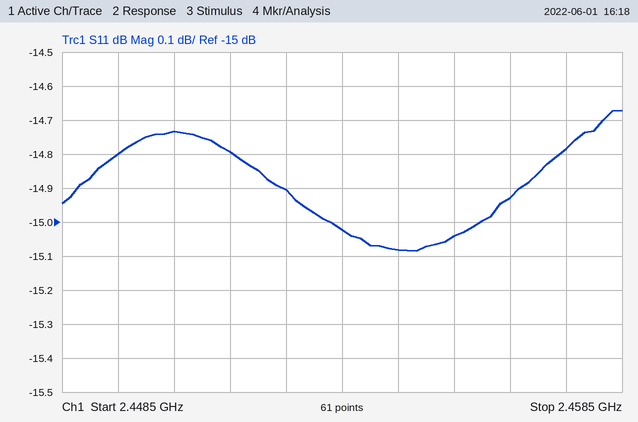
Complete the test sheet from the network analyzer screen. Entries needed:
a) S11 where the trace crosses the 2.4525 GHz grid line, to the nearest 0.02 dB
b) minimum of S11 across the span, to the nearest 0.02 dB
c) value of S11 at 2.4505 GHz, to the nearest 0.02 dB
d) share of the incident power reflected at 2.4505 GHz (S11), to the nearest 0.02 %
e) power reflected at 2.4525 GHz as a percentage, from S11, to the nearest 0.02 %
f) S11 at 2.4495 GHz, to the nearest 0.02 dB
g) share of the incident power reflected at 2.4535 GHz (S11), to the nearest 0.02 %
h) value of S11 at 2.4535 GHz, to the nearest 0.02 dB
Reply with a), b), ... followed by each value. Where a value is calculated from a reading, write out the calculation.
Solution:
a) -14.90 dB
b) -15.08 dB
c) -14.74 dB
d) 10^(-14.74/10) ≈ 3.36 %
e) 10^(-14.9/10) ≈ 3.24 %
f) -14.80 dB
g) 10^(-15.02/10) ≈ 3.15 %, so 3.14 % to the nearest 0.02 %
h) -15.02 dB
